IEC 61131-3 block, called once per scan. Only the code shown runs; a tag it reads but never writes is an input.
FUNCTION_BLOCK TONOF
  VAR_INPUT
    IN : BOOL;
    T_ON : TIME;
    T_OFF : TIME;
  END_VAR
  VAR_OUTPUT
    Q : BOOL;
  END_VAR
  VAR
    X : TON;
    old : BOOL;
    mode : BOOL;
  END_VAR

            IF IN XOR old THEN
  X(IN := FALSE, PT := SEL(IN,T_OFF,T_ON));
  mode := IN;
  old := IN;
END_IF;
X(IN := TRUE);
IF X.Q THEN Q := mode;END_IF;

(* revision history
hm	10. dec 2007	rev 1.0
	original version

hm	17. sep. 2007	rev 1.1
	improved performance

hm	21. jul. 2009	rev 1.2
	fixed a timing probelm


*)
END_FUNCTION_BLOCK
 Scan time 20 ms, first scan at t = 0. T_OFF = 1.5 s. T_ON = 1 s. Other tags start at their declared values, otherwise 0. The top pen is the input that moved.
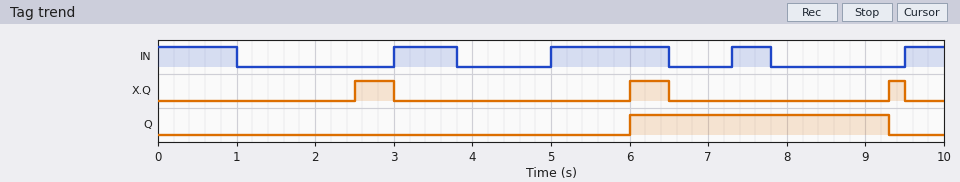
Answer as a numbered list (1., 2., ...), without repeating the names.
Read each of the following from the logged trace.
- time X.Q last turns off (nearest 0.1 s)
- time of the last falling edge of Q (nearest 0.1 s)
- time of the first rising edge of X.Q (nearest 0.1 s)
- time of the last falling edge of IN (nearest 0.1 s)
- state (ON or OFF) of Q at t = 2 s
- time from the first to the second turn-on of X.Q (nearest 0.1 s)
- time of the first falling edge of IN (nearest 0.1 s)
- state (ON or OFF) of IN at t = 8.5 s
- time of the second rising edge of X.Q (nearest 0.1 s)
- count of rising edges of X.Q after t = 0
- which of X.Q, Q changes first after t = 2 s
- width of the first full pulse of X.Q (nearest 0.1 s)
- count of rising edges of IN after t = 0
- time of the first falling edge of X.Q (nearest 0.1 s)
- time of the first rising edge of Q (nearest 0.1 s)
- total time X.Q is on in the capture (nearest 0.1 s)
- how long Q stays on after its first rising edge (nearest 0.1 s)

1. 9.5 s
2. 9.3 s
3. 2.5 s
4. 7.8 s
5. OFF
6. 3.5 s
7. 1.0 s
8. OFF
9. 6.0 s
10. 3
11. X.Q
12. 0.5 s
13. 4
14. 3.0 s
15. 6.0 s
16. 1.2 s
17. 3.3 s
